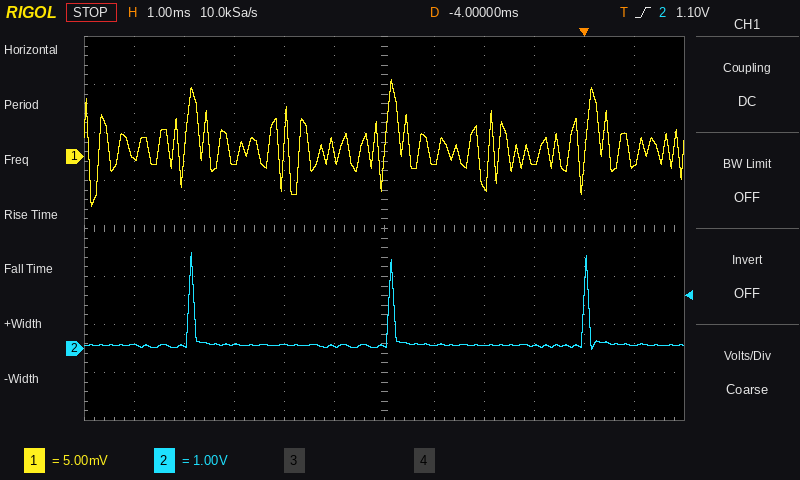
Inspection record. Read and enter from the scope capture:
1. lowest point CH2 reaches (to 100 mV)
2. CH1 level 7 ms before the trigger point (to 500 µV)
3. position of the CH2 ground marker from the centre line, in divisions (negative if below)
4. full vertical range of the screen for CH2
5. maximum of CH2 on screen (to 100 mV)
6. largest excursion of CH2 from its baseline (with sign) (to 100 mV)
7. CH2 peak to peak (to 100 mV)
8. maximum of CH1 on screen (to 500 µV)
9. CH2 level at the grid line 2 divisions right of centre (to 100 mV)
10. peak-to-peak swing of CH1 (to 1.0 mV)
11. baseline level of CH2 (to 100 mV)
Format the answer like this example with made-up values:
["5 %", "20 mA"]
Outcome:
["0.0 V", "-500 µV", "-2.5 div", "8 V", "2.0 V", "+1.9 V", "2.0 V", "8.0 mV", "100 mV", "13.0 mV", "100 mV"]
